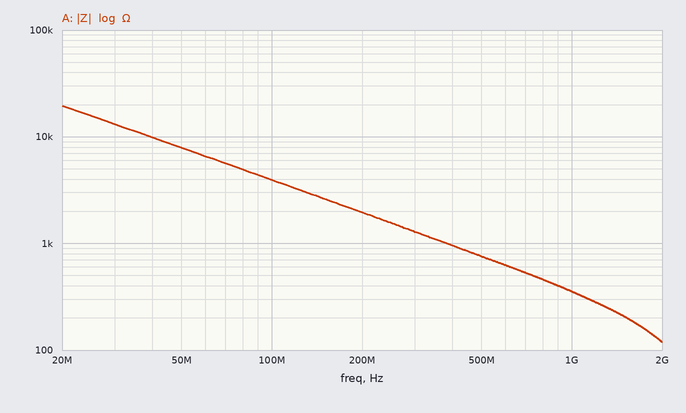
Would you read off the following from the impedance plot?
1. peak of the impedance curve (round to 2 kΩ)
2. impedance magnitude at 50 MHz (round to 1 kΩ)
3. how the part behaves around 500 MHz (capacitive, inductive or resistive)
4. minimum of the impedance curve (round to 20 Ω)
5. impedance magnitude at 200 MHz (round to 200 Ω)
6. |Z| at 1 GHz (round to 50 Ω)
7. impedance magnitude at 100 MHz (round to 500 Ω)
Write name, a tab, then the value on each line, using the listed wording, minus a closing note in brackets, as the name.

peak of the impedance curve	20 kΩ
impedance magnitude at 50 MHz	8 kΩ
how the part behaves around 500 MHz	capacitive
minimum of the impedance curve	120 Ω
impedance magnitude at 200 MHz	2.0 kΩ
|Z| at 1 GHz	350 Ω
impedance magnitude at 100 MHz	4.0 kΩ
